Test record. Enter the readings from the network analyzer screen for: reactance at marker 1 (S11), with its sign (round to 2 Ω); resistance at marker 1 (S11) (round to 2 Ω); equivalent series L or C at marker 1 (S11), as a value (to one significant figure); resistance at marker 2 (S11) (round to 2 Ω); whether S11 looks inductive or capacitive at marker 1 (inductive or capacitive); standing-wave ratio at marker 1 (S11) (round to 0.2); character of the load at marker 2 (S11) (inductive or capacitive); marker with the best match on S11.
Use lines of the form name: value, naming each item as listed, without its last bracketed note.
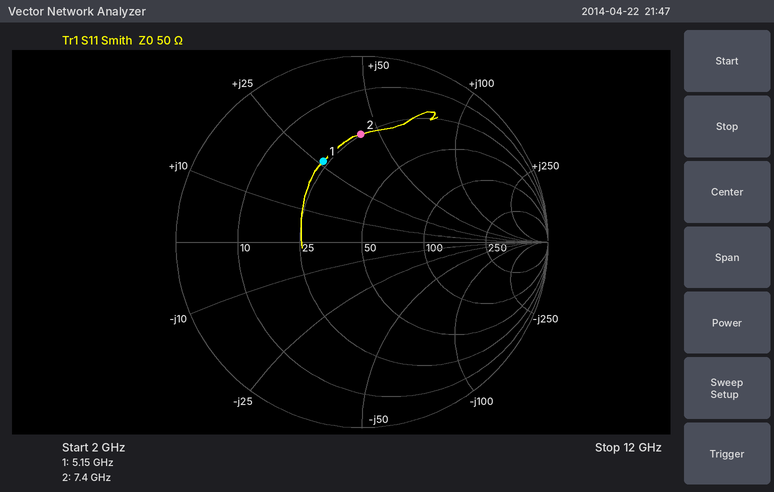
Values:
reactance at marker 1 (S11), with its sign: +26 Ω
resistance at marker 1 (S11): 24 Ω
equivalent series L or C at marker 1 (S11), as a value: 800 pH
resistance at marker 2 (S11): 24 Ω
whether S11 looks inductive or capacitive at marker 1: inductive
standing-wave ratio at marker 1 (S11): 2.8
character of the load at marker 2 (S11): inductive
marker with the best match on S11: marker 1
